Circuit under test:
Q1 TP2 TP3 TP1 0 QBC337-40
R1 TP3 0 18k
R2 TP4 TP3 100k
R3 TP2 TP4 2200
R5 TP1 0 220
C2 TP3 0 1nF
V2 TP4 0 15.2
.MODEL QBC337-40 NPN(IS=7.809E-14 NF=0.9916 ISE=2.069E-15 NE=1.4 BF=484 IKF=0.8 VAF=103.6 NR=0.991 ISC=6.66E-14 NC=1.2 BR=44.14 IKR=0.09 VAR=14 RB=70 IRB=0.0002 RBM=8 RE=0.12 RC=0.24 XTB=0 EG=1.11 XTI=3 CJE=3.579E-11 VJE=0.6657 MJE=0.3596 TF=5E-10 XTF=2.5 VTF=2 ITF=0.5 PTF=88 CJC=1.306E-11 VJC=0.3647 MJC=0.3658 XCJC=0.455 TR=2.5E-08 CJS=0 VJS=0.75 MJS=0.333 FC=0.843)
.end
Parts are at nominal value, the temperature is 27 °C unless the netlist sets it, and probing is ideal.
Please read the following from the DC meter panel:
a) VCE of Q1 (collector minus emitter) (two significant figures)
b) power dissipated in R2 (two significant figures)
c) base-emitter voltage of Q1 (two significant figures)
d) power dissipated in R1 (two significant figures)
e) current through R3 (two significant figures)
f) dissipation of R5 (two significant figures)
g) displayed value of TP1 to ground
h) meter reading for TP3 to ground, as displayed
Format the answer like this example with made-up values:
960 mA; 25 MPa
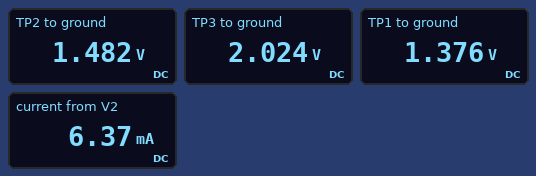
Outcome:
110 mV; 1.7 mW; 650 mV; 230 µW; 6.2 mA; 8.6 mW; 1.376 V; 2.024 V
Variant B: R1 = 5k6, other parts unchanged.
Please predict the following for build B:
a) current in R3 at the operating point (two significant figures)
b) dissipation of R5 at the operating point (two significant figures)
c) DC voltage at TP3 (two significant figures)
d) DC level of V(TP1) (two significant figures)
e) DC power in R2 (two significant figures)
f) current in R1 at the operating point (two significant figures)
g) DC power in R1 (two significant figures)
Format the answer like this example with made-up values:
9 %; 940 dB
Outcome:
920 µA; 190 µW; 800 mV; 200 mV; 2.1 mW; 140 µA; 110 µW
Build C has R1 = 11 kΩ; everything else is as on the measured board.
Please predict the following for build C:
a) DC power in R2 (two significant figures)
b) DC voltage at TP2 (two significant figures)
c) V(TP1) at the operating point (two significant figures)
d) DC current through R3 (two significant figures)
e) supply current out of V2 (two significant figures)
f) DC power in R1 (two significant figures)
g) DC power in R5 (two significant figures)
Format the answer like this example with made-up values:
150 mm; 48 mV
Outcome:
1.9 mW; 7.2 V; 800 mV; 3.6 mA; 3.8 mA; 190 µW; 2.9 mW
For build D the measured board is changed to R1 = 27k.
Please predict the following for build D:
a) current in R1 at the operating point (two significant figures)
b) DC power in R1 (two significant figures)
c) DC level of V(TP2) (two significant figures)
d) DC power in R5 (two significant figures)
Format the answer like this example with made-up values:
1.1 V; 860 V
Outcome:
76 µA; 150 µW; 1.4 V; 8.8 mW
